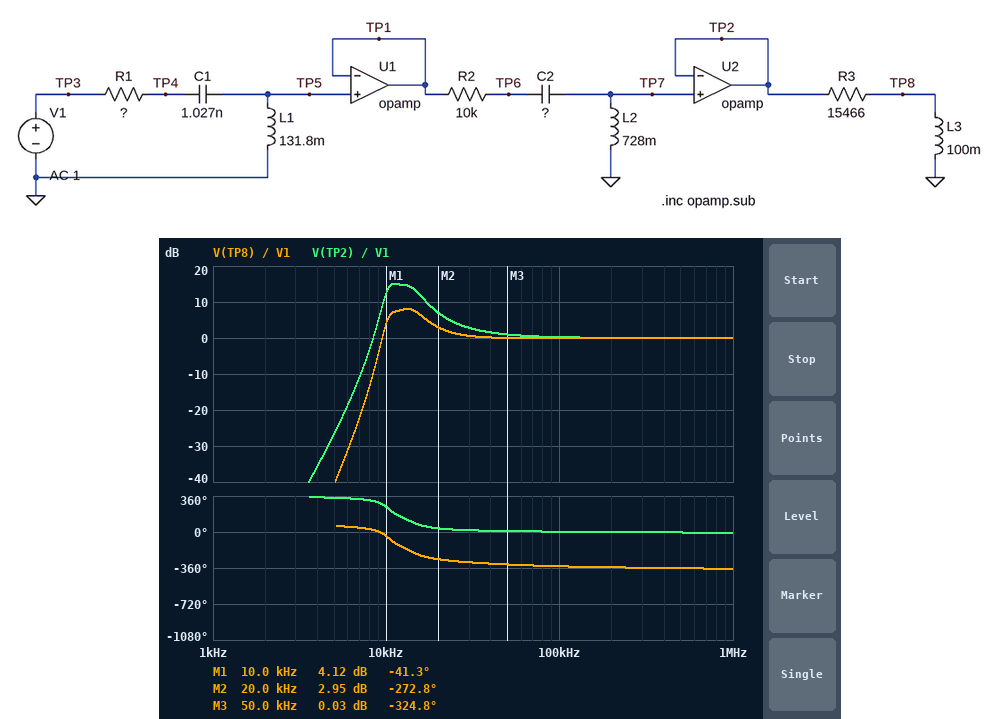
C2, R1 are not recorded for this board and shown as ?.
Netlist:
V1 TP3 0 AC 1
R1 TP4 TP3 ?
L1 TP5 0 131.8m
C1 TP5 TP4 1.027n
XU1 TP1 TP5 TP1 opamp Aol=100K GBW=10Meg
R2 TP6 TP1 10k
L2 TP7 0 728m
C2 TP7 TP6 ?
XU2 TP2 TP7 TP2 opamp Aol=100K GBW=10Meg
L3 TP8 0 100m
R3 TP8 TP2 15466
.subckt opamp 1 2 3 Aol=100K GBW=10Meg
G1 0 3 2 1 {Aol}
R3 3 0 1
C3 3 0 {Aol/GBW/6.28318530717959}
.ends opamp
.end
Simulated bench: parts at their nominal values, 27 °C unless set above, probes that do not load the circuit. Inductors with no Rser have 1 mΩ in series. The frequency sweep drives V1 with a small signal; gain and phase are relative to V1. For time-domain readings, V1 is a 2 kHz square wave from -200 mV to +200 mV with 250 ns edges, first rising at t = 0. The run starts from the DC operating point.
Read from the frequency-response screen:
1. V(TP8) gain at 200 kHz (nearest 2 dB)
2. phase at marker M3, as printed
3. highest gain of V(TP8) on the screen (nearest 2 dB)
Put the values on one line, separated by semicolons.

0 dB; -324.8 deg; 8 dB
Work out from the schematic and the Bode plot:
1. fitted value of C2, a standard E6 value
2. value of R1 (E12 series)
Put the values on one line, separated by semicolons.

330 pF; 4.7 kΩ
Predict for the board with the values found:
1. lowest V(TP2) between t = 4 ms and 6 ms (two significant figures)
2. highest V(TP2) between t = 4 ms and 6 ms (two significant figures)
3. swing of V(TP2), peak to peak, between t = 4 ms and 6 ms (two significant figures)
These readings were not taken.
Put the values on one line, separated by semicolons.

-430 mV; 430 mV; 850 mV
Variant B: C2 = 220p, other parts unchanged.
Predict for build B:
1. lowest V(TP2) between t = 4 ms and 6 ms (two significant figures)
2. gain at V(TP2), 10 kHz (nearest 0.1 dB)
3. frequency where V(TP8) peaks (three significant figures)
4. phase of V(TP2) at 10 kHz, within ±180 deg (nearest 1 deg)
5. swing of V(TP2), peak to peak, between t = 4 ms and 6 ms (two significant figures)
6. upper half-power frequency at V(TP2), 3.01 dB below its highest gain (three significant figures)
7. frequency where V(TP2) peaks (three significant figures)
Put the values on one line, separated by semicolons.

-600 mV; 3.8 dB; 13.0 kHz; -54 deg; 1.2 V; 14.4 kHz; 12.9 kHz
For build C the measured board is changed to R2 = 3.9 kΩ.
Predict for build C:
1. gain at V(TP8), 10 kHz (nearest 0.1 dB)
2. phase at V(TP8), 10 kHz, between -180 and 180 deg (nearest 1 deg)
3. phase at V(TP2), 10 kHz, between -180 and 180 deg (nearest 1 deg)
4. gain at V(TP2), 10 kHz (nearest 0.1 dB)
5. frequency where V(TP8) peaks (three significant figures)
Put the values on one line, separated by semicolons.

11.1 dB; -23 deg; -91 deg; 19.6 dB; 10.4 kHz
